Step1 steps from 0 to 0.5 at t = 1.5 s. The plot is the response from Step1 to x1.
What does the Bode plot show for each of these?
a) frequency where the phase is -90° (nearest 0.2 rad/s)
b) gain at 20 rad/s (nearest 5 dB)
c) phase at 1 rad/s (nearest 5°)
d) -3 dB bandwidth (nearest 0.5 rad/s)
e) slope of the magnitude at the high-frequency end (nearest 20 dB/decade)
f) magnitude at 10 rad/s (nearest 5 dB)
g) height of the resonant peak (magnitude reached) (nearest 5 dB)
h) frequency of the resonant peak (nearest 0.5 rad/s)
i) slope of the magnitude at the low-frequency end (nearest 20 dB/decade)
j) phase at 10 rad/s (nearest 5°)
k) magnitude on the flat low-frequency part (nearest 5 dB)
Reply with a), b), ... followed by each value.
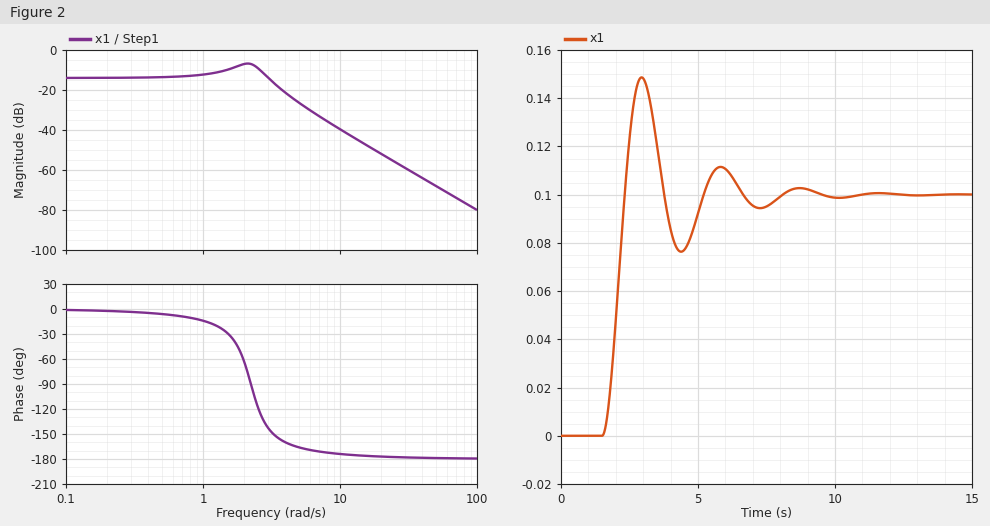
a) 2.2 rad/s
b) -50 dB
c) -15°
d) 3.5 rad/s
e) -40 dB/decade
f) -40 dB
g) -5 dB
h) 2.0 rad/s
i) 0 dB/decade
j) -175°
k) -15 dB
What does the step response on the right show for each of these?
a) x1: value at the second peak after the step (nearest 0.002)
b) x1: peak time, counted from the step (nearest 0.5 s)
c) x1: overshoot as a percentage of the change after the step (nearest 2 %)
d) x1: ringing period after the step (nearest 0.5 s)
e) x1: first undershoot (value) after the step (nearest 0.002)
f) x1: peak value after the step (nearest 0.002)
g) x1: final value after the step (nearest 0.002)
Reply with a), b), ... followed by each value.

a) 0.112
b) 1.5 s
c) 48 %
d) 3.0 s
e) 0.076
f) 0.148
g) 0.100
